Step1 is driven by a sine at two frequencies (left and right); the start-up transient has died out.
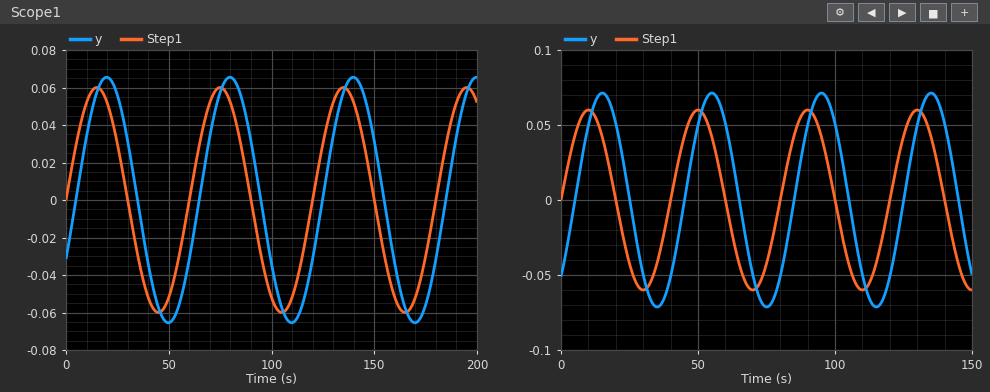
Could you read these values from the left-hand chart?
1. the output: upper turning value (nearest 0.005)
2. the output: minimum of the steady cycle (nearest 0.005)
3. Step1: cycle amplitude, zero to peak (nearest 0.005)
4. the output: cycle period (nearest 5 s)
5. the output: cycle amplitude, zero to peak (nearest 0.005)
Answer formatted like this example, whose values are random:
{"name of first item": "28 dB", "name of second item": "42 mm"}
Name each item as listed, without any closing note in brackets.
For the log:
{"the output: upper turning value": "0.065", "the output: minimum of the steady cycle": "-0.065", "Step1: cycle amplitude, zero to peak": "0.060", "the output: cycle period": "60 s", "the output: cycle amplitude, zero to peak": "0.065"}
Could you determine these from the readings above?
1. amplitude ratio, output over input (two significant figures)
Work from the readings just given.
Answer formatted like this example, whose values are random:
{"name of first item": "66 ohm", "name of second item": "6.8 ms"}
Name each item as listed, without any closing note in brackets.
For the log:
{"amplitude ratio, output over input": "1.1"}
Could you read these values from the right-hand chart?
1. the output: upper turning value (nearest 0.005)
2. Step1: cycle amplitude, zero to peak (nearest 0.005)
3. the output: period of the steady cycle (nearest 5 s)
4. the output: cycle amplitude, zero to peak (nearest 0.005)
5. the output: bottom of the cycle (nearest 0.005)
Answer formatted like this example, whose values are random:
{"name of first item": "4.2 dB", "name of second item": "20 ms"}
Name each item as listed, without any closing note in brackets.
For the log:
{"the output: upper turning value": "0.070", "Step1: cycle amplitude, zero to peak": "0.060", "the output: period of the steady cycle": "40 s", "the output: cycle amplitude, zero to peak": "0.070", "the output: bottom of the cycle": "-0.070"}
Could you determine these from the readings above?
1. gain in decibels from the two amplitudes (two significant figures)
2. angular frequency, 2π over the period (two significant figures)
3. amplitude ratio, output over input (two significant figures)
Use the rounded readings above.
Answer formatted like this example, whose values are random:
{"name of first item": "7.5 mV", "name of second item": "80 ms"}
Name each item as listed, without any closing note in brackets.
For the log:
{"gain in decibels from the two amplitudes": "1.3 dB", "angular frequency, 2π over the period": "0.16 rad/s", "amplitude ratio, output over input": "1.2"}
